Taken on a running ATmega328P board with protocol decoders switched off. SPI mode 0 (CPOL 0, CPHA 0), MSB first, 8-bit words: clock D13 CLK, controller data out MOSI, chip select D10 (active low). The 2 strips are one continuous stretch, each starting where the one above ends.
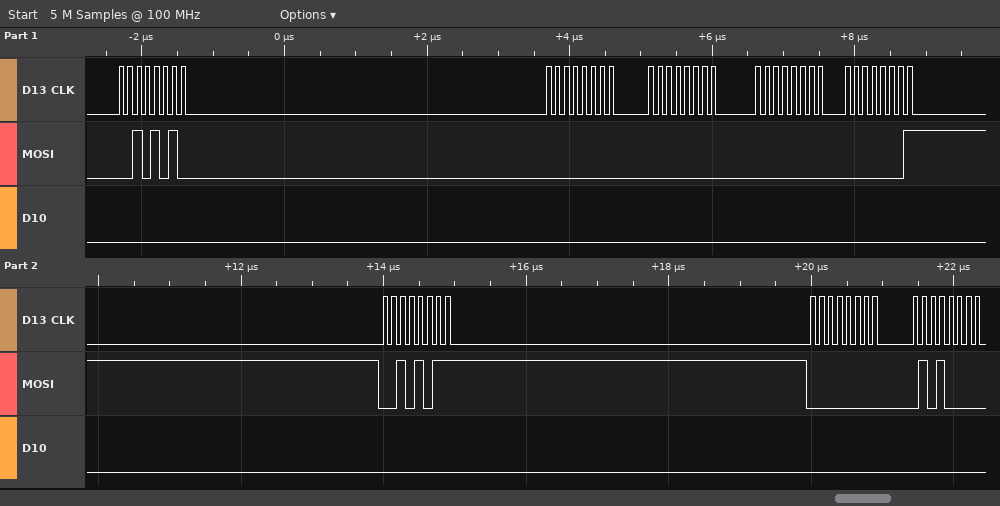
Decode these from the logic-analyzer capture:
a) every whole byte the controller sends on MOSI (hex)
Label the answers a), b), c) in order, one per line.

a) 2A 00 00 00 01 2B 00 50
